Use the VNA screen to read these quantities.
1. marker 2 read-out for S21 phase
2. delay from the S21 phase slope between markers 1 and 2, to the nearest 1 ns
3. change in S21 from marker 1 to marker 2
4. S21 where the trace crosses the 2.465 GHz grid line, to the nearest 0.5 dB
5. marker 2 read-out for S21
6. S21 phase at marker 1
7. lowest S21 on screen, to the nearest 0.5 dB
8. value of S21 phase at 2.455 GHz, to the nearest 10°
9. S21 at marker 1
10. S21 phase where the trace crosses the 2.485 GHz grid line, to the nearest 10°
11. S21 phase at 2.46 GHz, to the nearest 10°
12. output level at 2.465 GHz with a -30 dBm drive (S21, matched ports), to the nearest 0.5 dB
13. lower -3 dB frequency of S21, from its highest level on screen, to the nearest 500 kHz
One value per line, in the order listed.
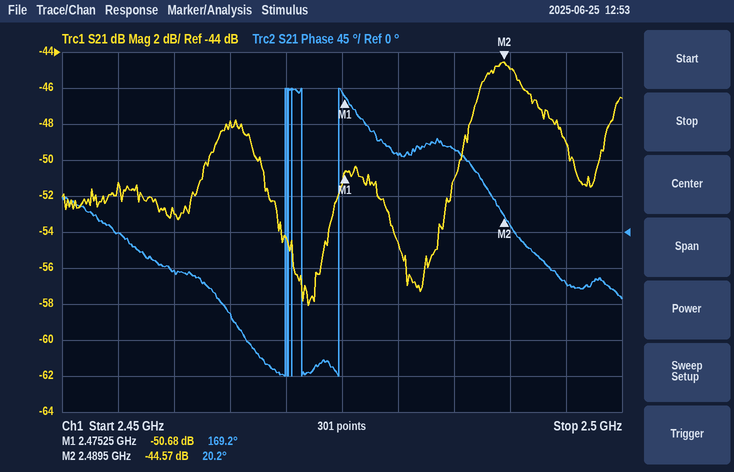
20.2°
29 ns
6.11 dB
-48.0 dB
-44.57 dB
169.2°
-58.0 dB
0°
-50.68 dB
100°
-50°
-78.0 dBm
2.4865 GHz
